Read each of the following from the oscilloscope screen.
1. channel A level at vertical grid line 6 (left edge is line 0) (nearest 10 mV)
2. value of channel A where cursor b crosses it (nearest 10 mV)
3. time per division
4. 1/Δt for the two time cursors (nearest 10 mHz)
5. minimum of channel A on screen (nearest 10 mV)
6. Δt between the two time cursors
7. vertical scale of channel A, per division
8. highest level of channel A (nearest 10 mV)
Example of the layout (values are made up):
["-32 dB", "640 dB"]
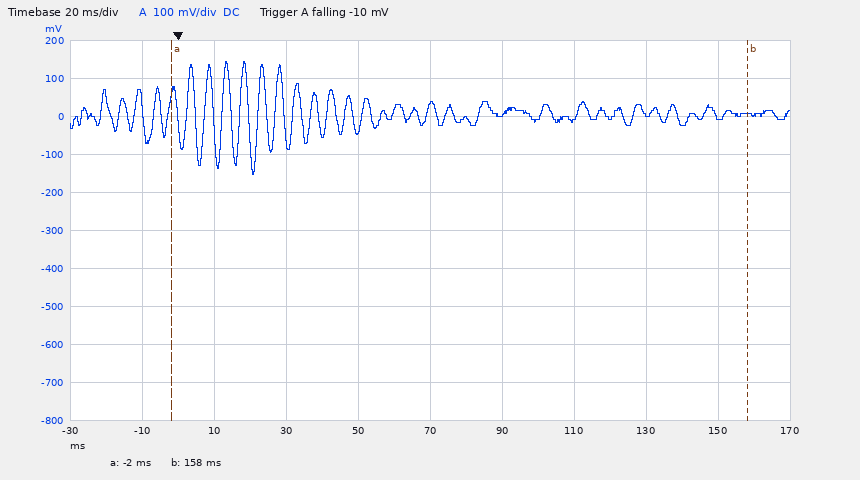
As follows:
["10 mV", "10 mV", "20 ms", "6.25 Hz", "-150 mV", "160 ms", "100 mV", "140 mV"]
